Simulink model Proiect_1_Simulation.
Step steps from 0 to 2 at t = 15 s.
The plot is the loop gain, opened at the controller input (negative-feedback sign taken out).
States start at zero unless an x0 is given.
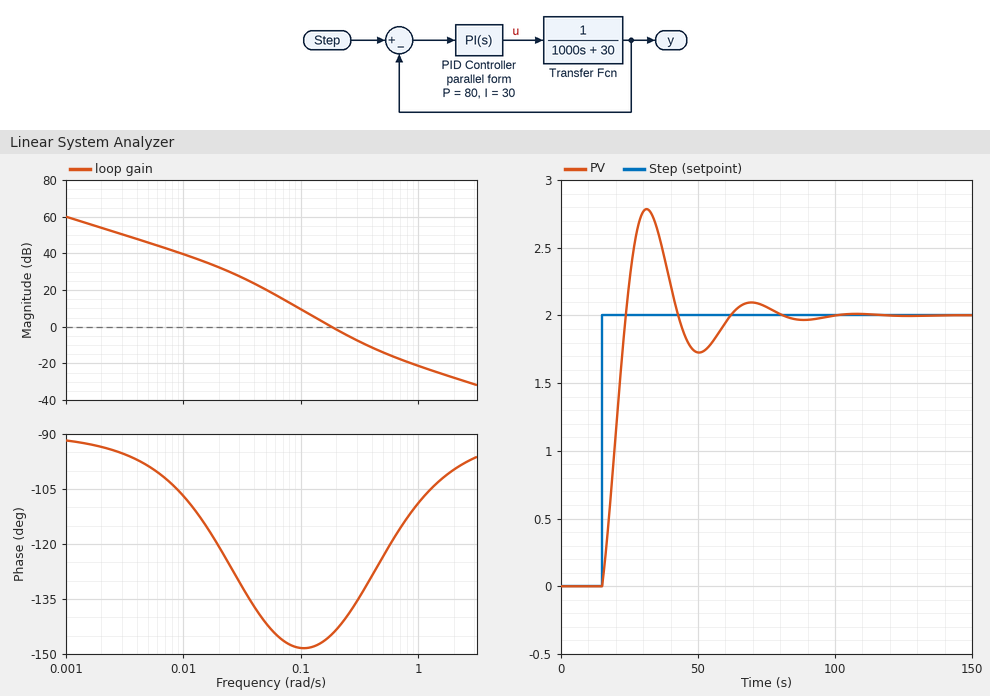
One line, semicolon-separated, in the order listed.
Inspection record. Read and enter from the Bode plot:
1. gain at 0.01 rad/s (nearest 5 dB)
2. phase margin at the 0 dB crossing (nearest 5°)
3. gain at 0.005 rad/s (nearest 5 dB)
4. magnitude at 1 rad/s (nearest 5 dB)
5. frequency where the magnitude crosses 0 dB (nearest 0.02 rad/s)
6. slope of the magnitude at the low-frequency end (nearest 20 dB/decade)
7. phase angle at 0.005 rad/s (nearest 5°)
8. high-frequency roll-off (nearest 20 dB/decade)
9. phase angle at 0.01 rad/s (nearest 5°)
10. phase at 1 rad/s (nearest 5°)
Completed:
40 dB; 35°; 45 dB; -20 dB; 0.18 rad/s; -20 dB/decade; -100°; -20 dB/decade; -105°; -110°
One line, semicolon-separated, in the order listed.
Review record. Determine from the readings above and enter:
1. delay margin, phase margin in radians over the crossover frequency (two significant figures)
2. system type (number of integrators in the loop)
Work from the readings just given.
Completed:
3.4 s; 1
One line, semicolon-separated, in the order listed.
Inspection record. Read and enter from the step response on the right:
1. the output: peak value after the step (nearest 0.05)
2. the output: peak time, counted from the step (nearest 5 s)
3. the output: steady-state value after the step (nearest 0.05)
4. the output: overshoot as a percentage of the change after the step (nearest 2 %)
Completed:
2.80; 15 s; 2.00; 40 %
